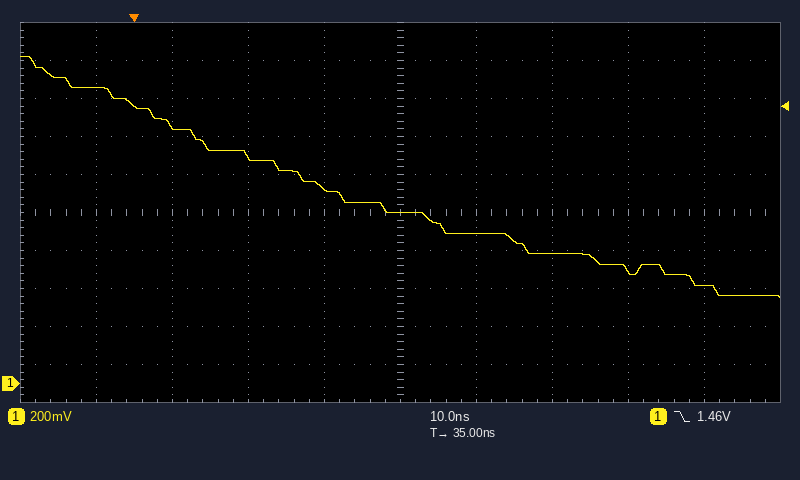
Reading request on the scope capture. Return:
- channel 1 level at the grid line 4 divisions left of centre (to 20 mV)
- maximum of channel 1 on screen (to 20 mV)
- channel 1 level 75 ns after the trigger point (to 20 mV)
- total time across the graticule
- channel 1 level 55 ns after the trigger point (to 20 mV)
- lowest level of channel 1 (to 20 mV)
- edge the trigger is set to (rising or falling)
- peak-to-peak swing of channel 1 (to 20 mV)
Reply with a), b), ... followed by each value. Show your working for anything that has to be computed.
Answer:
a) 1.56 V
b) 1.72 V
c) 520 mV
d) 100 ns
e) 680 mV
f) 460 mV
g) falling
h) 1.72 V − (460 mV) = 1.26 V
